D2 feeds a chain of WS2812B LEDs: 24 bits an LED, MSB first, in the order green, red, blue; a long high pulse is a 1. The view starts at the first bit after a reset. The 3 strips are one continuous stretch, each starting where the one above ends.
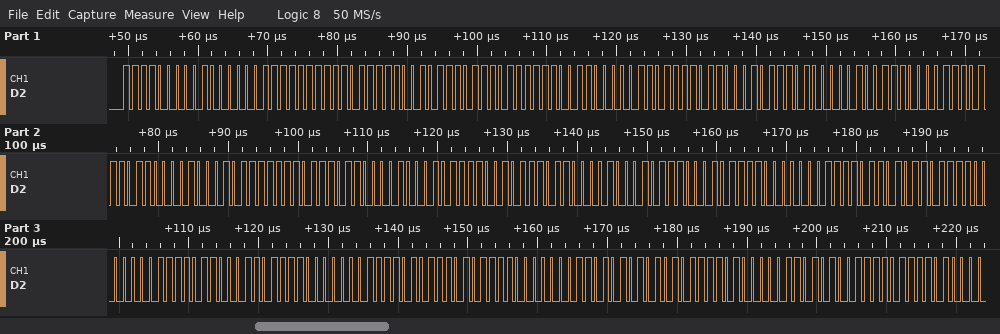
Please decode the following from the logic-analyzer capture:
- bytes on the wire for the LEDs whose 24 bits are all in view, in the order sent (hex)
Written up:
F0 40 FF DF 2E EF CC 1B D8 BA 09 C3 BB 08 BF BB 08 BC BB 08 B8 BC 07 B5 BC 07 B1 BC 07 AE BC 06 AA BD 06 A7
